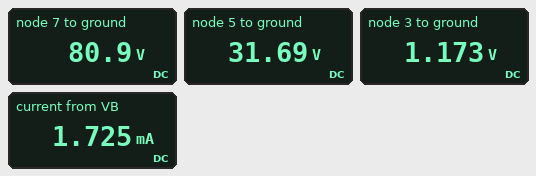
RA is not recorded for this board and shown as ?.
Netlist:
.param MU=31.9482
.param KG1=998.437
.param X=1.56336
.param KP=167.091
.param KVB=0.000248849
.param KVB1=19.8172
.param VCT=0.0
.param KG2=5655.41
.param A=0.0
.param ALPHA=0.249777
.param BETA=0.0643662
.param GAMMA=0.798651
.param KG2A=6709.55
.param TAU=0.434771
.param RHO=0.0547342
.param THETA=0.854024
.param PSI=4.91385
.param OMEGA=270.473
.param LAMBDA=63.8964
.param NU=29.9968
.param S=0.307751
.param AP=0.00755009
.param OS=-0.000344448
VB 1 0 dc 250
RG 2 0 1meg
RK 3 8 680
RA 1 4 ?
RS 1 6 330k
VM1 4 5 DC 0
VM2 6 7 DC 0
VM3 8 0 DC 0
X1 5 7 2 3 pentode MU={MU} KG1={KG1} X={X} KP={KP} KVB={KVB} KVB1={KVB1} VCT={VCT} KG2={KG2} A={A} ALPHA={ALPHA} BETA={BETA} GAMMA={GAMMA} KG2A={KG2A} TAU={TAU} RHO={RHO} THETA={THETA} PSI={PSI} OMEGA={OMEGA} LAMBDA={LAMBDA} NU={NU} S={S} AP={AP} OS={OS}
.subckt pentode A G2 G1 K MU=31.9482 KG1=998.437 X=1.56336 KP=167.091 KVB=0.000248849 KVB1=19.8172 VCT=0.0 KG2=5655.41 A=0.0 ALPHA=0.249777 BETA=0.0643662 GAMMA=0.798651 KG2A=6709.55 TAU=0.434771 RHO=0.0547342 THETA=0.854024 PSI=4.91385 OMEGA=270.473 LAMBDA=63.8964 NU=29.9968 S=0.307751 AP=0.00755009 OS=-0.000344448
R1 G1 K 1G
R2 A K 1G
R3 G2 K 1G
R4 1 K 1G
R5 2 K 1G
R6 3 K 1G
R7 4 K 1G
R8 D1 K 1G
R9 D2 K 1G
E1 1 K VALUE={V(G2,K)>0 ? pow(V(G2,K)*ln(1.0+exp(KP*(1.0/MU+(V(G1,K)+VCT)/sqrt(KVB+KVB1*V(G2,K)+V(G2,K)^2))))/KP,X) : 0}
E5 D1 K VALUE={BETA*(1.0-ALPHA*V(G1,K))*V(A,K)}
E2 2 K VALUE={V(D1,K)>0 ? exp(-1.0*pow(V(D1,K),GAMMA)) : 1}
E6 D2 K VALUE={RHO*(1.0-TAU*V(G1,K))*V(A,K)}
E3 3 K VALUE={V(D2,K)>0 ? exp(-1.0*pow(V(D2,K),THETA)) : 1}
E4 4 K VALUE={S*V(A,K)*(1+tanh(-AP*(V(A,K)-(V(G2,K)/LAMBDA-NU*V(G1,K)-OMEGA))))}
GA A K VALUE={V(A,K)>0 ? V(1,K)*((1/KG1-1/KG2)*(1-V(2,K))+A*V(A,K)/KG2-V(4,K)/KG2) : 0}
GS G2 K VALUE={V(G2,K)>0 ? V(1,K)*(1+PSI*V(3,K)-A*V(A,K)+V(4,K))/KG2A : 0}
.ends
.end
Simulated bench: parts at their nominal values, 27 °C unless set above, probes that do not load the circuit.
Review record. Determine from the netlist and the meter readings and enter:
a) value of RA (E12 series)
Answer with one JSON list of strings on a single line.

["180 kΩ"]
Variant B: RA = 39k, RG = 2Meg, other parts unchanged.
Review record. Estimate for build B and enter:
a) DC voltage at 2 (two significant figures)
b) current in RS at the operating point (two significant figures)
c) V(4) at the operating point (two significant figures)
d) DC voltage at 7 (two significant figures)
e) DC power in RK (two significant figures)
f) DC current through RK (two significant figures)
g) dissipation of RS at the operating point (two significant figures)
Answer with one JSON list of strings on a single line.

["3.1 mV", "450 µA", "180 V", "100 V", "3.6 mW", "2.3 mA", "67 mW"]
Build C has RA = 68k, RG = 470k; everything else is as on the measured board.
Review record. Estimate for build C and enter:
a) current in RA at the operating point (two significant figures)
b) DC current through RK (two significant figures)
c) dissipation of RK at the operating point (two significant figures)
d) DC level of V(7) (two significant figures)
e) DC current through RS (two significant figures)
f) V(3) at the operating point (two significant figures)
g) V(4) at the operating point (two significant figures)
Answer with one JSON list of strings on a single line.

["1.7 mA", "2.2 mA", "3.2 mW", "97 V", "460 µA", "1.5 V", "130 V"]
